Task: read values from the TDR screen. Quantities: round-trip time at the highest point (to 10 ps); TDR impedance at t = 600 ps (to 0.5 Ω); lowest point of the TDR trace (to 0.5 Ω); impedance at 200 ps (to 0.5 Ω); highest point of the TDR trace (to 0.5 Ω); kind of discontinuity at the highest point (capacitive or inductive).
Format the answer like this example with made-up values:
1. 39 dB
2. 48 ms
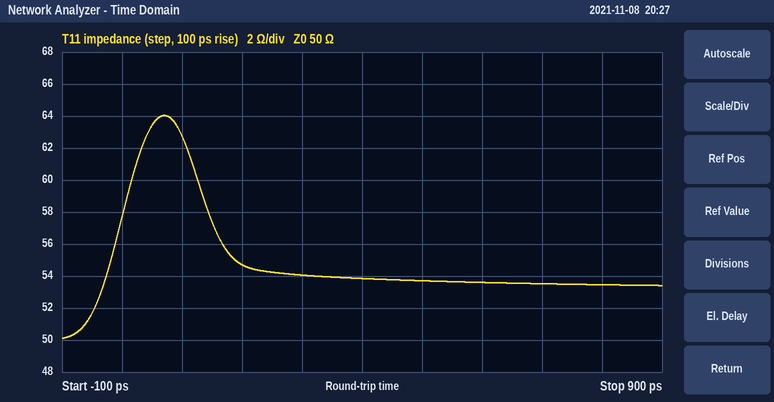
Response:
1. 70 ps
2. 53.5 Ω
3. 50.0 Ω
4. 54.5 Ω
5. 64.0 Ω
6. inductive
